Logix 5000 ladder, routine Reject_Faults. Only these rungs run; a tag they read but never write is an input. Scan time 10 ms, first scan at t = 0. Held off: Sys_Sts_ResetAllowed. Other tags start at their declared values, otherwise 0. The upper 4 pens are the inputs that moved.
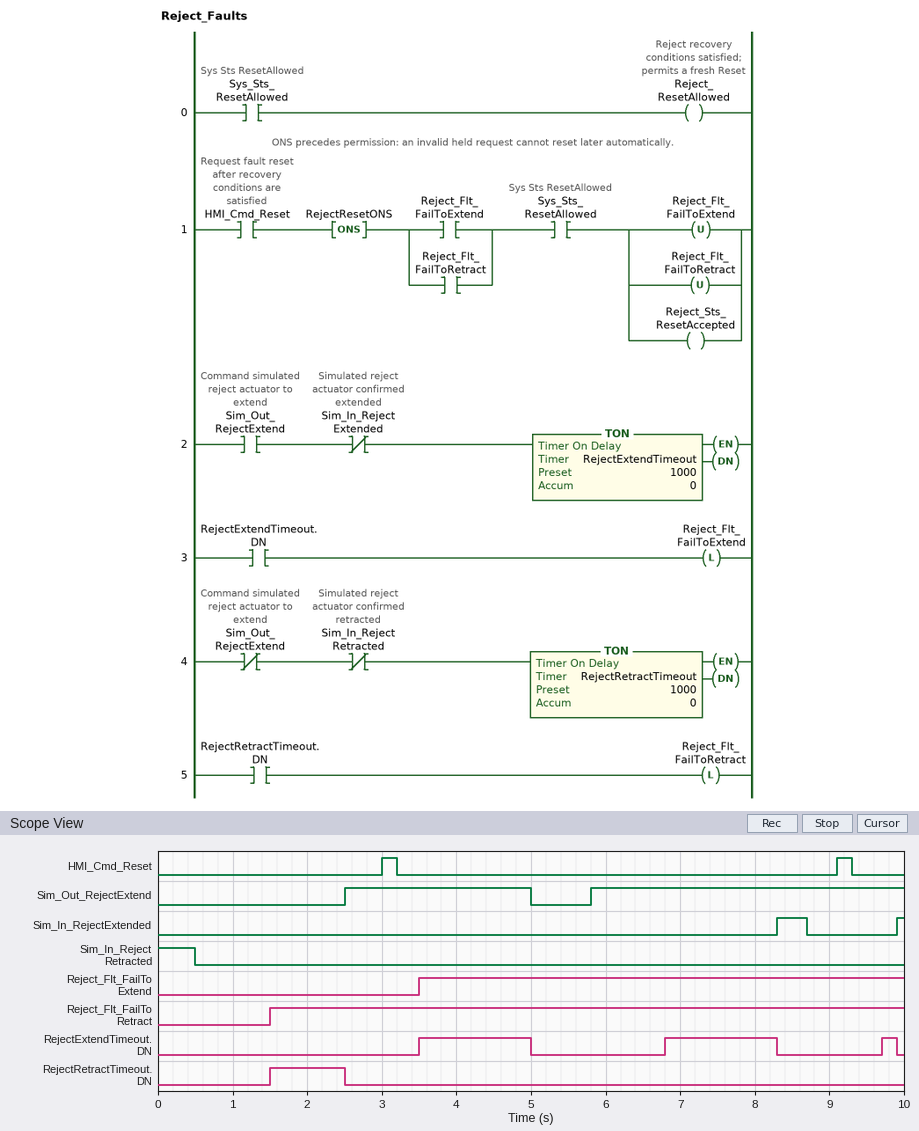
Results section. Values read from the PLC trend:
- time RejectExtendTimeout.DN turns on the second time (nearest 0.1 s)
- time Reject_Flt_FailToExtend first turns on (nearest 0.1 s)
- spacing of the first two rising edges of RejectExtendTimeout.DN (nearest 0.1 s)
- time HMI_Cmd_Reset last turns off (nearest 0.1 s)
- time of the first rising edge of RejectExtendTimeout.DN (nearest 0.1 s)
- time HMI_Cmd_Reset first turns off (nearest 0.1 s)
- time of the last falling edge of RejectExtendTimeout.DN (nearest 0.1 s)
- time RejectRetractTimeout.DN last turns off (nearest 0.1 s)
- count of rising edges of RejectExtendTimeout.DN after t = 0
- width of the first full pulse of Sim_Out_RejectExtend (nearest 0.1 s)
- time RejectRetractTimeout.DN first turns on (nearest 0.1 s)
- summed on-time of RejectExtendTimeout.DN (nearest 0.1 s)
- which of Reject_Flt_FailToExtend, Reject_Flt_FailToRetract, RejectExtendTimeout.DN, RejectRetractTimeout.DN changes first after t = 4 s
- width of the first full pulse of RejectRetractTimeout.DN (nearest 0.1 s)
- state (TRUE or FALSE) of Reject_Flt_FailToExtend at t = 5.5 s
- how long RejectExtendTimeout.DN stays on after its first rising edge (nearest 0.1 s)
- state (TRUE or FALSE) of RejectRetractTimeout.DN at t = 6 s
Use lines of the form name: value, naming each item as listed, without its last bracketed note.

time RejectExtendTimeout.DN turns on the second time: 6.8 s
time Reject_Flt_FailToExtend first turns on: 3.5 s
spacing of the first two rising edges of RejectExtendTimeout.DN: 3.3 s
time HMI_Cmd_Reset last turns off: 9.3 s
time of the first rising edge of RejectExtendTimeout.DN: 3.5 s
time HMI_Cmd_Reset first turns off: 3.2 s
time of the last falling edge of RejectExtendTimeout.DN: 9.9 s
time RejectRetractTimeout.DN last turns off: 2.5 s
count of rising edges of RejectExtendTimeout.DN after t = 0: 3
width of the first full pulse of Sim_Out_RejectExtend: 2.5 s
time RejectRetractTimeout.DN first turns on: 1.5 s
summed on-time of RejectExtendTimeout.DN: 3.2 s
which of Reject_Flt_FailToExtend, Reject_Flt_FailToRetract, RejectExtendTimeout.DN, RejectRetractTimeout.DN changes first after t = 4 s: RejectExtendTimeout.DN
width of the first full pulse of RejectRetractTimeout.DN: 1.0 s
state (TRUE or FALSE) of Reject_Flt_FailToExtend at t = 5.5 s: TRUE
how long RejectExtendTimeout.DN stays on after its first rising edge: 1.5 s
state (TRUE or FALSE) of RejectRetractTimeout.DN at t = 6 s: FALSE
